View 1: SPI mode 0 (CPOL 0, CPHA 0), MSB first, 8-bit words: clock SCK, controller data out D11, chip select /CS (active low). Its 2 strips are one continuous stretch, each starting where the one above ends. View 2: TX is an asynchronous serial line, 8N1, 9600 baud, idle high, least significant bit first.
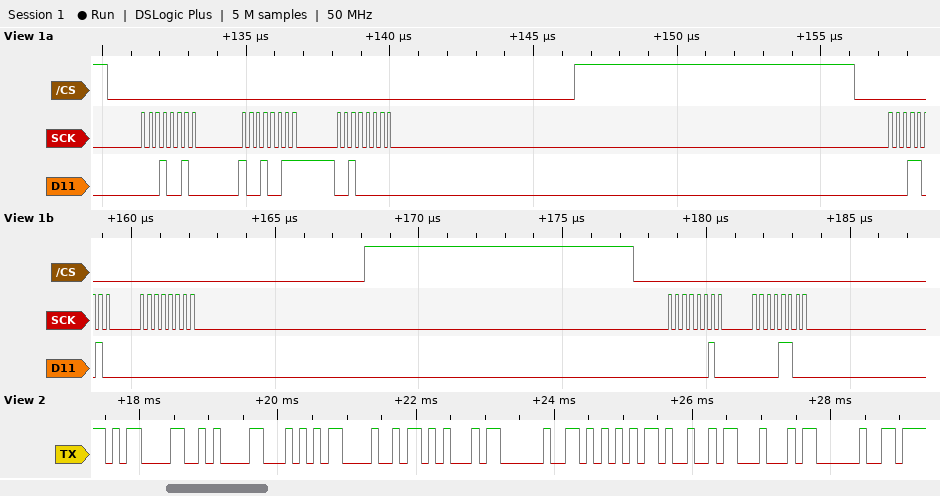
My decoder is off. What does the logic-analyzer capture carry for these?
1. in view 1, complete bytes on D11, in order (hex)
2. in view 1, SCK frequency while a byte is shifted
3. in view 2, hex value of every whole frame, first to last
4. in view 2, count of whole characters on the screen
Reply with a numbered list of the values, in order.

1. 12 93 20 1A 00 02 0C
2. 4 MHz
3. 0D 0A 54 48 45 20 55 49 44 20
4. 10
